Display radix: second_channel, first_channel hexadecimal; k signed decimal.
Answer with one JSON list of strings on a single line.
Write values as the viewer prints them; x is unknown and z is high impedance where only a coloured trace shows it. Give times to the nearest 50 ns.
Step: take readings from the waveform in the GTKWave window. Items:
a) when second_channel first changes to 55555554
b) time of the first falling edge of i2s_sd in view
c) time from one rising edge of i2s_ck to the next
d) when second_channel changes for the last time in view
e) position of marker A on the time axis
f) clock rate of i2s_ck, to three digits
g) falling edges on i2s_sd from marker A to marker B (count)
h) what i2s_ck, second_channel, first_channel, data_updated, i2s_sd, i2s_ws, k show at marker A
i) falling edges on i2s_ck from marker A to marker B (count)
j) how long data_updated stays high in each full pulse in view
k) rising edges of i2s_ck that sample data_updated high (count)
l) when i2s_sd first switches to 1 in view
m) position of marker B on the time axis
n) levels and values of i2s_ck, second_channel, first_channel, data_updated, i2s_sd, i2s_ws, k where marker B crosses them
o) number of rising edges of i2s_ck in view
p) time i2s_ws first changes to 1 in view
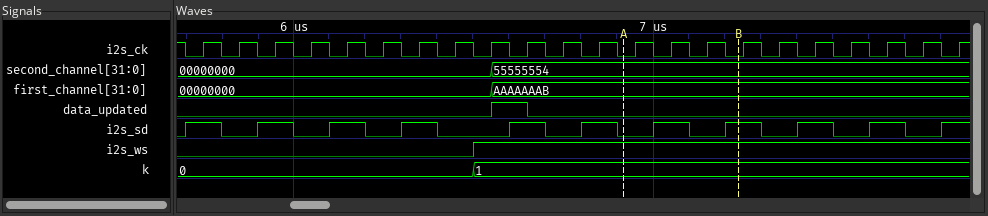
["6550 ns", "5800 ns", "100 ns", "6550 ns", "6900 ns", "10.0 MHz", "1", "i2s_ck=0, second_channel=55555554, first_channel=AAAAAAAB, data_updated=0, i2s_sd=0, i2s_ws=1, k=1", "3", "100 ns", "1", "5700 ns", "7250 ns", "i2s_ck=0, second_channel=55555554, first_channel=AAAAAAAB, data_updated=0, i2s_sd=1, i2s_ws=1, k=1", "22", "6500 ns"]
